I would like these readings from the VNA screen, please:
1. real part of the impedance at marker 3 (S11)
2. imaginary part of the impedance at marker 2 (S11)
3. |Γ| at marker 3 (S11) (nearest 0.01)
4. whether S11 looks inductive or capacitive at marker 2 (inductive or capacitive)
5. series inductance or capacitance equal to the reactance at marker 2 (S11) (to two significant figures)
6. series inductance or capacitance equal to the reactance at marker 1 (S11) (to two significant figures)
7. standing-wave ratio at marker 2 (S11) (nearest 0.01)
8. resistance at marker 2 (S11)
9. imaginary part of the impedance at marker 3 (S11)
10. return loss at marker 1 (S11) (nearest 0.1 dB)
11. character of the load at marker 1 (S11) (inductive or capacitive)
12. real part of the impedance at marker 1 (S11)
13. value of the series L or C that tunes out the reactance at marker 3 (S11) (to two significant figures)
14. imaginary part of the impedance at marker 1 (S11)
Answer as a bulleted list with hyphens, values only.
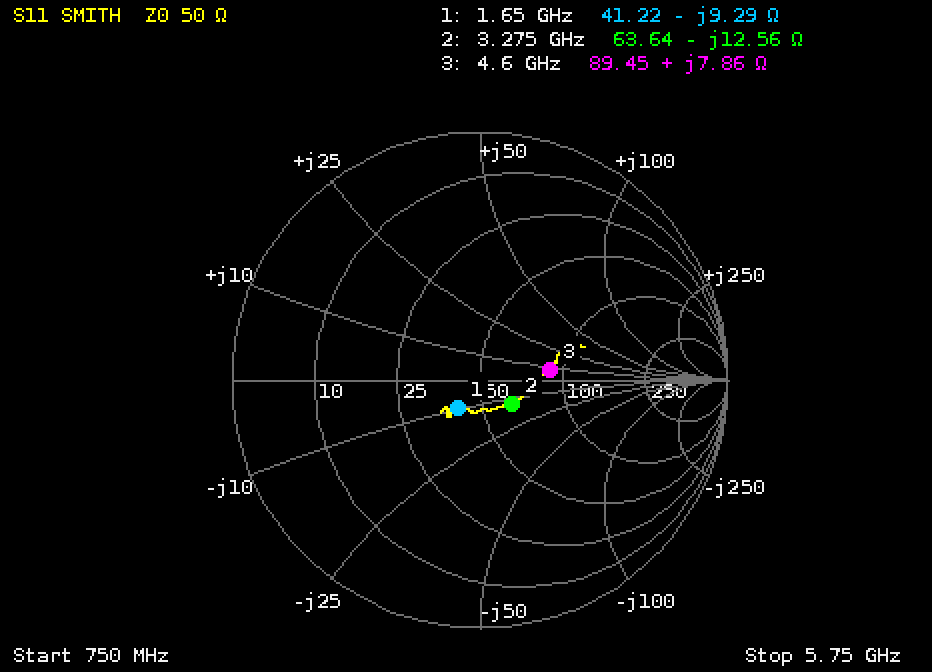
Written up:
- 89.45 Ω
- -12.56 Ω
- 0.29
- capacitive
- 3.9 pF
- 10 pF
- 1.39
- 63.64 Ω
- +7.86 Ω
- 17.1 dB
- capacitive
- 41.22 Ω
- 4.4 pF
- -9.29 Ω
